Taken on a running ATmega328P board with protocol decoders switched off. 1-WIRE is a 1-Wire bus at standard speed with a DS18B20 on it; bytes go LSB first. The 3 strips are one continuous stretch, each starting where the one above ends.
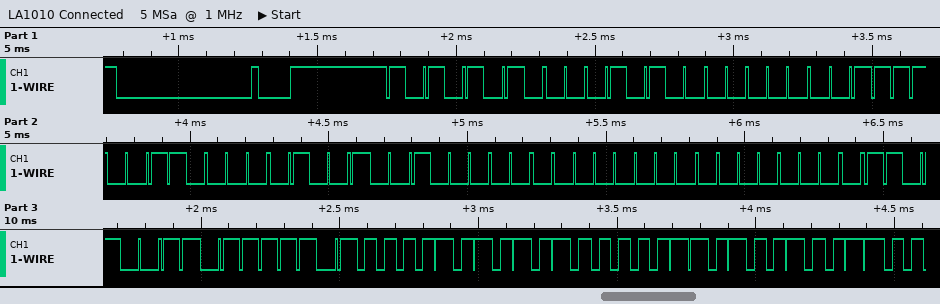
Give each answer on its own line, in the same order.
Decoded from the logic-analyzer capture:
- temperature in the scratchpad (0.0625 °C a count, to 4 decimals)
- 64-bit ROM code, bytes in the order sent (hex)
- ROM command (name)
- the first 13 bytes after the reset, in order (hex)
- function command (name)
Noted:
85.0000 °C
28 80 67 90 04 00 00 CB
Match ROM
55 28 80 67 90 04 00 00 CB BE 50 05 4B
Read Scratchpad
